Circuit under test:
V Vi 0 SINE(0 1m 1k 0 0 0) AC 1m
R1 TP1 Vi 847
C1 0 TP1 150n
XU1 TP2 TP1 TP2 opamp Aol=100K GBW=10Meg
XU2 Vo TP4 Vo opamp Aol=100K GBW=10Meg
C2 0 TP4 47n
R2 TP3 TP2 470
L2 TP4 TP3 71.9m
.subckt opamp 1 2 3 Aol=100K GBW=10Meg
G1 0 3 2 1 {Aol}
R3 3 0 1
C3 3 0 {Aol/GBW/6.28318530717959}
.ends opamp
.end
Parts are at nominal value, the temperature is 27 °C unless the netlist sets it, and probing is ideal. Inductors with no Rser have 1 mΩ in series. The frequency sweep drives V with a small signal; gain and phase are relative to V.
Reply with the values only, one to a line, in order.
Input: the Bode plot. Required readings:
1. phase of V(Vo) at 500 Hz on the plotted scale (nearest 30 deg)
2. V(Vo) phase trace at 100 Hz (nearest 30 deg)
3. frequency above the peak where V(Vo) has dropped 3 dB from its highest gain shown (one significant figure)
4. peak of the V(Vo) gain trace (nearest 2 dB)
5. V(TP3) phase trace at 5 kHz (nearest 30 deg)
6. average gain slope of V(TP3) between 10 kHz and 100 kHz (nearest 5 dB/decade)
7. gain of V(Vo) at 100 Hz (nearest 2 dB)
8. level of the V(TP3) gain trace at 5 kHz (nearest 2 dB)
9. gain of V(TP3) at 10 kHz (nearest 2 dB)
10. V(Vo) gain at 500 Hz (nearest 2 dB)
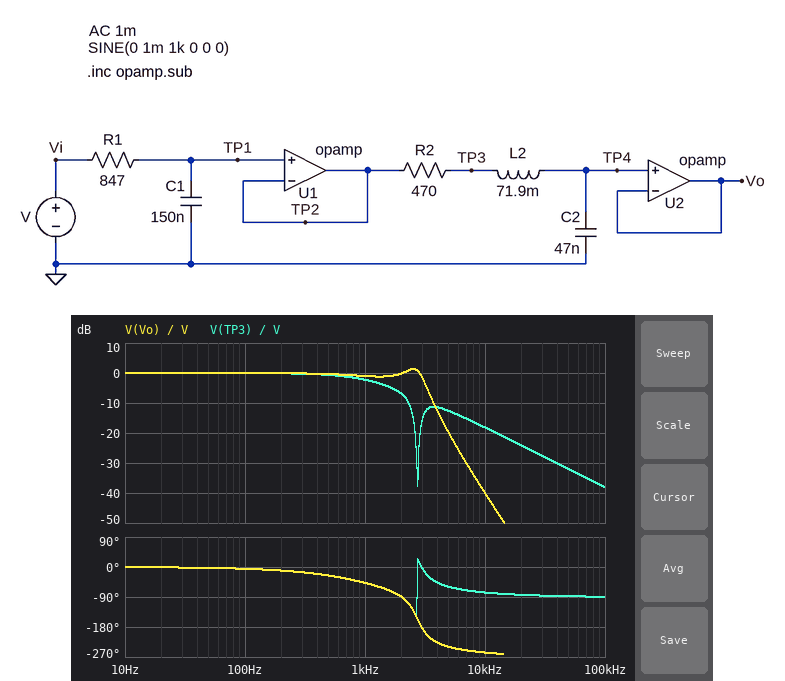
-30 deg
0 deg
3 kHz
2 dB
-60 deg
-20 dB/decade
0 dB
-12 dB
-18 dB
0 dB
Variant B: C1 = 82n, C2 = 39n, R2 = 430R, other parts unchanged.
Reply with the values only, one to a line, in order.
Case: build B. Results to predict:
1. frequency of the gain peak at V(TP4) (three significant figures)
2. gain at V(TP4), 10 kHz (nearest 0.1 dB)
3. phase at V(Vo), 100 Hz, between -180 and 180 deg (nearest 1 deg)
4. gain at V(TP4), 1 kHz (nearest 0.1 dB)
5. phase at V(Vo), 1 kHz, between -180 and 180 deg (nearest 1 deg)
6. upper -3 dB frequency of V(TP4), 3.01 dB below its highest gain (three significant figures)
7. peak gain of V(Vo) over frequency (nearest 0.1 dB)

2.88 kHz
-33.1 dB
-3 deg
0.2 dB
-30 deg
3.31 kHz
5.9 dB
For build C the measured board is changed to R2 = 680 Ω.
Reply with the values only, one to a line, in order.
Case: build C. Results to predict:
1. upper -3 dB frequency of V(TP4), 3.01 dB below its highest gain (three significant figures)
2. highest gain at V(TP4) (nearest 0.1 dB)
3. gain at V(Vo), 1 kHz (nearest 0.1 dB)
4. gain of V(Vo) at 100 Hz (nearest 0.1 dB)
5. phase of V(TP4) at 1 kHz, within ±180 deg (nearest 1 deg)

2.83 kHz
0 dB
-1.1 dB
0 dB
-52 deg
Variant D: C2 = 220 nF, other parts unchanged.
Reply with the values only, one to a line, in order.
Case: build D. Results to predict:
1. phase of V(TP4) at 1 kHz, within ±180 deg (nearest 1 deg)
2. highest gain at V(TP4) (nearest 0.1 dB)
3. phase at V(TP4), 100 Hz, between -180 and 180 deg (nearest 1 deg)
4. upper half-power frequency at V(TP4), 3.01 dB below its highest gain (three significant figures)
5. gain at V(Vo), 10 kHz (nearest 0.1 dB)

-99 deg
0.5 dB
-8 deg
1.36 kHz
-53.9 dB
